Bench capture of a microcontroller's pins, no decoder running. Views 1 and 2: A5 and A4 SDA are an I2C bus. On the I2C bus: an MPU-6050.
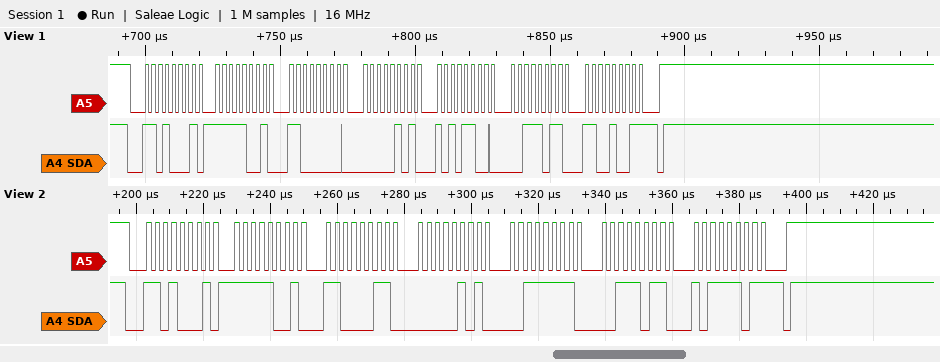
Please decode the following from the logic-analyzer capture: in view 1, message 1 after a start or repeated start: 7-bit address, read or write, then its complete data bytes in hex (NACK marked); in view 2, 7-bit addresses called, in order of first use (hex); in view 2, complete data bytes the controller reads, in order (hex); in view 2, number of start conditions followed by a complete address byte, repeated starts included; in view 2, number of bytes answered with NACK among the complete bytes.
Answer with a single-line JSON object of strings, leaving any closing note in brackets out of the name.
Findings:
{"in view 1, message 1 after a start or repeated start: 7-bit address, read or write, then its complete data bytes in hex": "0x68 read: F9 C0 05 AC 3B C9 NACK", "in view 2, 7-bit addresses called, in order of first use": "0x68", "in view 2, complete data bytes the controller reads, in order": "F9 C3 05 3F 3B BD", "in view 2, number of start conditions followed by a complete address byte, repeated starts included": "1", "in view 2, number of bytes answered with NACK among the complete bytes": "1"}
